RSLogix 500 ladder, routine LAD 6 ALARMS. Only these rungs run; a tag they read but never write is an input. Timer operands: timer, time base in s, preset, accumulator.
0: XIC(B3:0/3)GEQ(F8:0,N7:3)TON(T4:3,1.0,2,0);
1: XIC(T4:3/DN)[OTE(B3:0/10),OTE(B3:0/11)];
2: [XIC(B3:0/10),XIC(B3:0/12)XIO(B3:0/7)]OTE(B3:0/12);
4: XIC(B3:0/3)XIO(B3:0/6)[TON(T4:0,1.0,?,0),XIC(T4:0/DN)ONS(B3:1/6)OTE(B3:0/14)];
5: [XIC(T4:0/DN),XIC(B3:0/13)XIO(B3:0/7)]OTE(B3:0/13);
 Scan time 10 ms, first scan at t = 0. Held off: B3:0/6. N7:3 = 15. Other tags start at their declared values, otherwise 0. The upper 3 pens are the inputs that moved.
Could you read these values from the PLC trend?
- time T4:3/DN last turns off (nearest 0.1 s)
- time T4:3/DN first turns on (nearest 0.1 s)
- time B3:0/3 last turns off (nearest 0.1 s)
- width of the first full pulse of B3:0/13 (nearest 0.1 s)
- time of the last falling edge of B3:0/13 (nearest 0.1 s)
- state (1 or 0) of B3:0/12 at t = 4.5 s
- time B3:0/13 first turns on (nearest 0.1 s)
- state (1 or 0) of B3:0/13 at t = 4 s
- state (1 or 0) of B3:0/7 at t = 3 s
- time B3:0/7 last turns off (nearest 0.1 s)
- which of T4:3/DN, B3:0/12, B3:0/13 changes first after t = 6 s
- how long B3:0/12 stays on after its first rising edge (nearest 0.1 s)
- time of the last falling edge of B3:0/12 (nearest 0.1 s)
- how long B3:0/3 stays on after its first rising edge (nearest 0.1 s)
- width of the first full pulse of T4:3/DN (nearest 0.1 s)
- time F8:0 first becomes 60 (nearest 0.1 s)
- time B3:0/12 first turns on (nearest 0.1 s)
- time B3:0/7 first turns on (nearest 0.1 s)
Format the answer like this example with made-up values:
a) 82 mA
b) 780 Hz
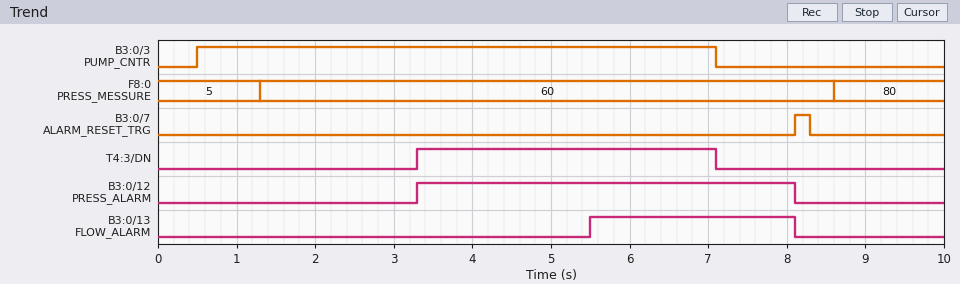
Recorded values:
a) 7.1 s
b) 3.3 s
c) 7.1 s
d) 2.6 s
e) 8.1 s
f) 1
g) 5.5 s
h) 0
i) 0
j) 8.3 s
k) T4:3/DN
l) 4.8 s
m) 8.1 s
n) 6.6 s
o) 3.8 s
p) 1.3 s
q) 3.3 s
r) 8.1 s
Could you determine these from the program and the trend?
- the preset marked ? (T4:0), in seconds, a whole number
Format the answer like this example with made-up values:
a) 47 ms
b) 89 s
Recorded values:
a) 5 s
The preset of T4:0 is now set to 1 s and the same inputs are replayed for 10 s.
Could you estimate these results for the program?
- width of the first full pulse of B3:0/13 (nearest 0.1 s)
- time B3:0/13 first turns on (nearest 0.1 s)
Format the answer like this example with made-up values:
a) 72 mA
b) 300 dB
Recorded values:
a) 6.6 s
b) 1.5 s
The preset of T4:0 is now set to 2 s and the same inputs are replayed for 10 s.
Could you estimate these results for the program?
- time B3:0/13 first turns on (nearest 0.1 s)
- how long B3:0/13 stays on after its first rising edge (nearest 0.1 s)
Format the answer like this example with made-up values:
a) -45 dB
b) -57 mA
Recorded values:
a) 2.5 s
b) 5.6 s
